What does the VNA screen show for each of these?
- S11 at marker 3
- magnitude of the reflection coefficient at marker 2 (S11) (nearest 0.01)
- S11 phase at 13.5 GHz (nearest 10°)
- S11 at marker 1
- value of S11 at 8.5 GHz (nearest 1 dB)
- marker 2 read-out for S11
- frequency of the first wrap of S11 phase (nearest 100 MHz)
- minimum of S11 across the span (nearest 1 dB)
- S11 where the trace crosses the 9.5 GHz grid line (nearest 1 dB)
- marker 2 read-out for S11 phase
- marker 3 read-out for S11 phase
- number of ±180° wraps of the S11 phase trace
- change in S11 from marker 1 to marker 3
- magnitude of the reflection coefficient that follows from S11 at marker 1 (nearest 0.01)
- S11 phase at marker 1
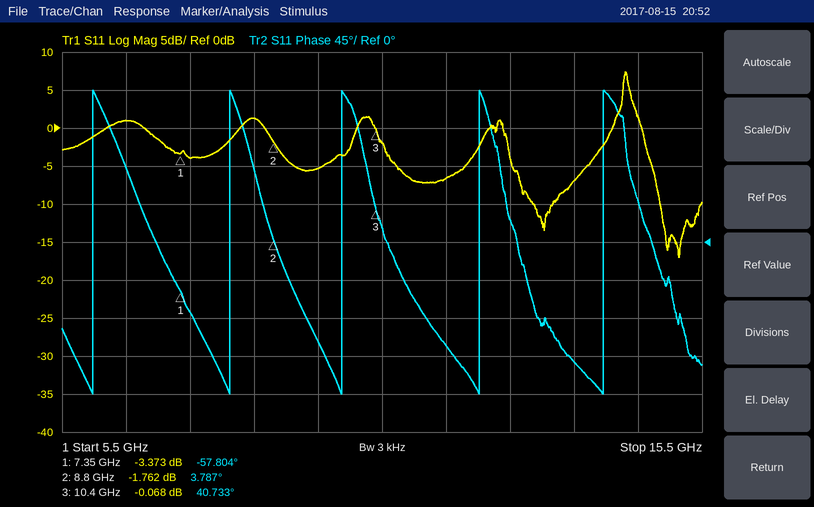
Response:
-0.068 dB
0.82
-140°
-3.373 dB
1 dB
-1.762 dB
6.0 GHz
-17 dB
-5 dB
3.787°
40.733°
5
3.305 dB
0.68
-57.804°
